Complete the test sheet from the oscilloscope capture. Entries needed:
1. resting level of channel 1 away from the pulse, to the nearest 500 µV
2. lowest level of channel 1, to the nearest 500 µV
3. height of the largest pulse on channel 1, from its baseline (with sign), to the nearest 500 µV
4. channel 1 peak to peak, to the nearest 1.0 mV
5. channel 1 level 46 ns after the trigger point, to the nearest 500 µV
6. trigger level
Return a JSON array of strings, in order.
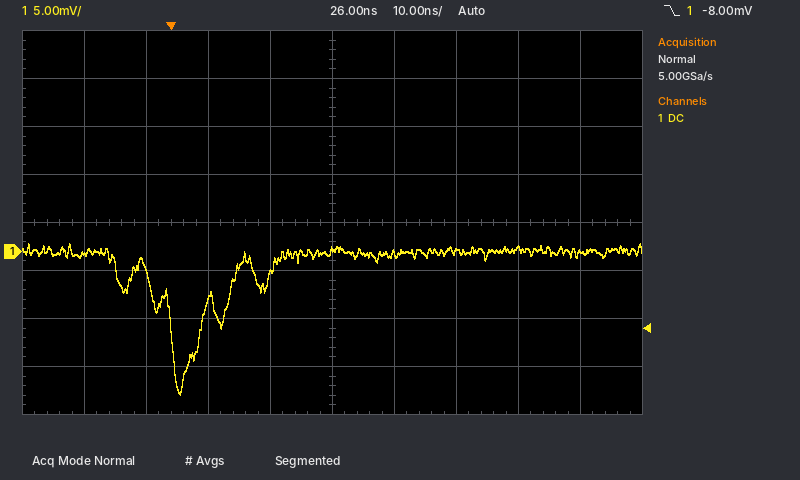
["0.0 mV", "-15.0 mV", "-15.0 mV", "16.0 mV", "0.0 mV", "-8.00 mV"]
